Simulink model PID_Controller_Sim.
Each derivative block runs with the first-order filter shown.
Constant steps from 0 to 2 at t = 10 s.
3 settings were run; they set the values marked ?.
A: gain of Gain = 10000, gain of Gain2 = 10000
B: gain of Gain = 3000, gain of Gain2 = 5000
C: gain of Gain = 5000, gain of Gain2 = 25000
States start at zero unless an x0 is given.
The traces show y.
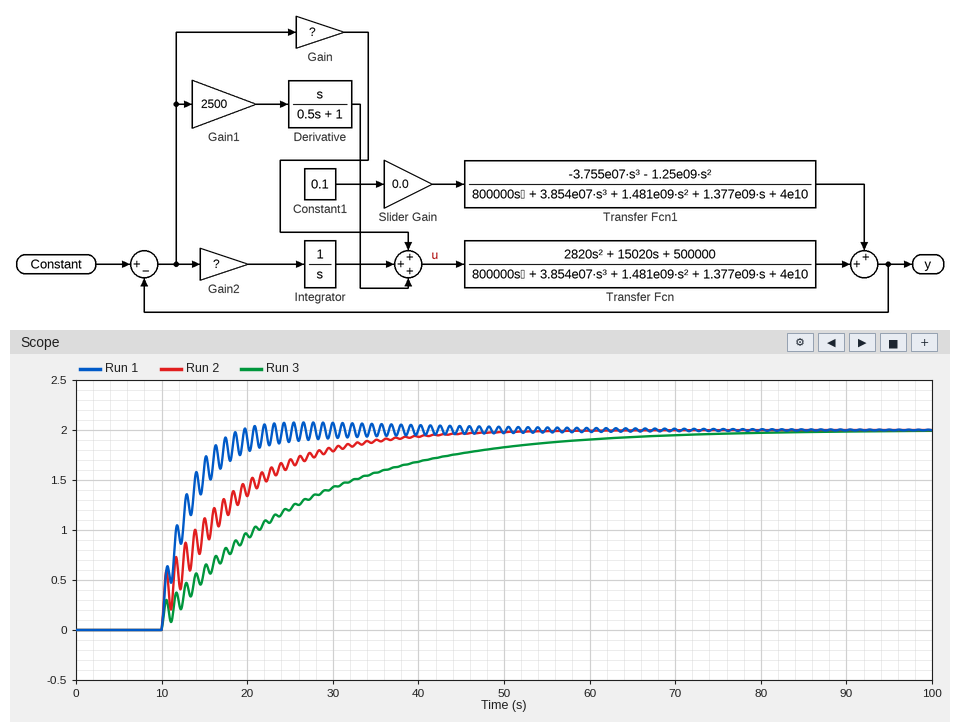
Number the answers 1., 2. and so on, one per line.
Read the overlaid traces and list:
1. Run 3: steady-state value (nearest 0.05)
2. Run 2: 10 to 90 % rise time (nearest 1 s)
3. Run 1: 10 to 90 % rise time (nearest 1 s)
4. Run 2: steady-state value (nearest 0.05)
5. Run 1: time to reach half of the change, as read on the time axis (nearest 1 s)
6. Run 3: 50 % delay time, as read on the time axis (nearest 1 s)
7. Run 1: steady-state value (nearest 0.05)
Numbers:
1. 2.00
2. 19 s
3. 6 s
4. 2.00
5. 12 s
6. 21 s
7. 2.00
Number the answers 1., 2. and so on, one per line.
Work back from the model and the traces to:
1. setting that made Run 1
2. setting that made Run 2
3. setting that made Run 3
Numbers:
1. C
2. A
3. B
